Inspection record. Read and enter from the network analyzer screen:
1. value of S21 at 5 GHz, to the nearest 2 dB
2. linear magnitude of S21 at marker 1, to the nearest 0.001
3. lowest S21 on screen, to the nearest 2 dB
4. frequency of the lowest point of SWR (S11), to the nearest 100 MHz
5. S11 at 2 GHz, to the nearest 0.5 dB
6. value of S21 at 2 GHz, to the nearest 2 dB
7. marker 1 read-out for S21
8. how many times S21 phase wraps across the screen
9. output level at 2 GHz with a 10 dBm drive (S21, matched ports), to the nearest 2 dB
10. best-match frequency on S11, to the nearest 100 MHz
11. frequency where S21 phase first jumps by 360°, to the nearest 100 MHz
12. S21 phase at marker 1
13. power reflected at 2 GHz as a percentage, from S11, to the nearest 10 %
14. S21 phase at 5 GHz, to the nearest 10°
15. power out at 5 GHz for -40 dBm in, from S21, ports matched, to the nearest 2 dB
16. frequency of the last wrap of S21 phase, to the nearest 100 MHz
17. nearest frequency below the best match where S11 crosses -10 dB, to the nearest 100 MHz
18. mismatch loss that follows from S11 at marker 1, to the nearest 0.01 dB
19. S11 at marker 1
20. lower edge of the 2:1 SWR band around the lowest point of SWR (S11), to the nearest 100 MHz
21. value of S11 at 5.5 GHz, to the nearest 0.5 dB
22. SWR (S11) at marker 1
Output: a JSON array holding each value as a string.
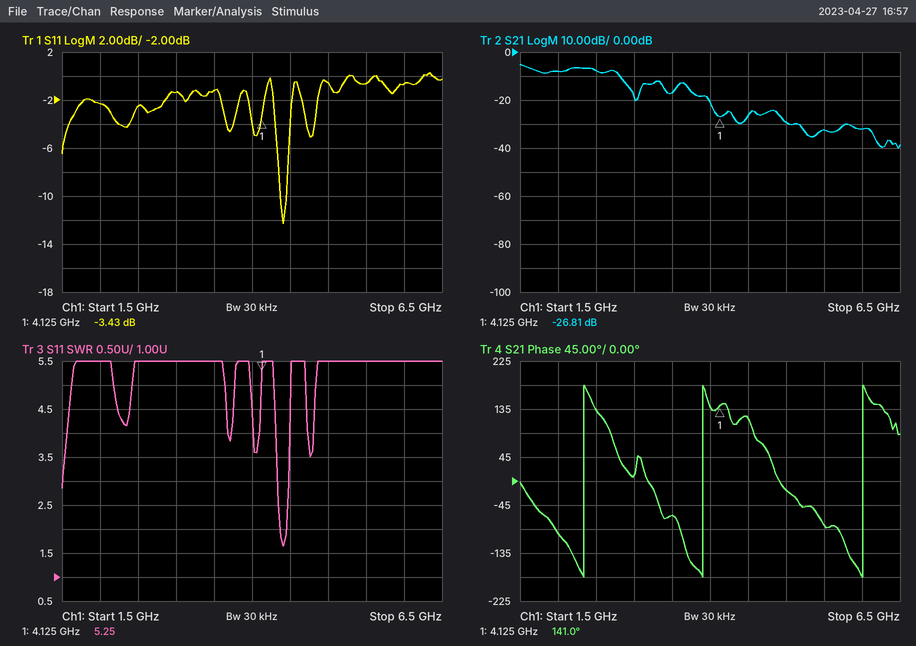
["-30 dB", "0.046", "-40 dB", "4.4 GHz", "-2.5 dB", "-8 dB", "-26.81 dB", "3", "2 dBm", "4.4 GHz", "2.3 GHz", "141.0°", "60 %", "-20°", "-70 dBm", "6.0 GHz", "4.4 GHz", "2.63 dB", "-3.43 dB", "4.4 GHz", "-0.5 dB", "5.25"]
